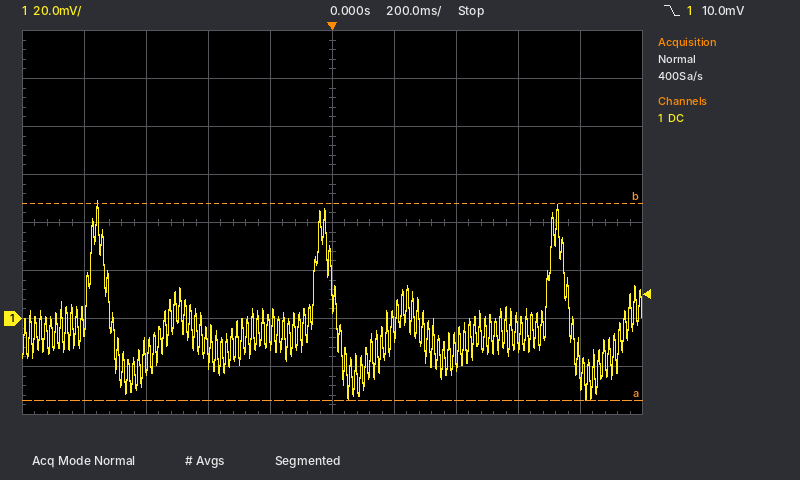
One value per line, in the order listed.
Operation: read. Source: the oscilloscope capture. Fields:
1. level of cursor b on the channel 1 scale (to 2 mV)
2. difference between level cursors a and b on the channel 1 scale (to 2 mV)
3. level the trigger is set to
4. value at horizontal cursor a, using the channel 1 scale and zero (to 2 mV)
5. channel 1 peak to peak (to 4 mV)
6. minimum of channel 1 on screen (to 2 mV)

48 mV
82 mV
10.0 mV
-34 mV
84 mV
-34 mV
